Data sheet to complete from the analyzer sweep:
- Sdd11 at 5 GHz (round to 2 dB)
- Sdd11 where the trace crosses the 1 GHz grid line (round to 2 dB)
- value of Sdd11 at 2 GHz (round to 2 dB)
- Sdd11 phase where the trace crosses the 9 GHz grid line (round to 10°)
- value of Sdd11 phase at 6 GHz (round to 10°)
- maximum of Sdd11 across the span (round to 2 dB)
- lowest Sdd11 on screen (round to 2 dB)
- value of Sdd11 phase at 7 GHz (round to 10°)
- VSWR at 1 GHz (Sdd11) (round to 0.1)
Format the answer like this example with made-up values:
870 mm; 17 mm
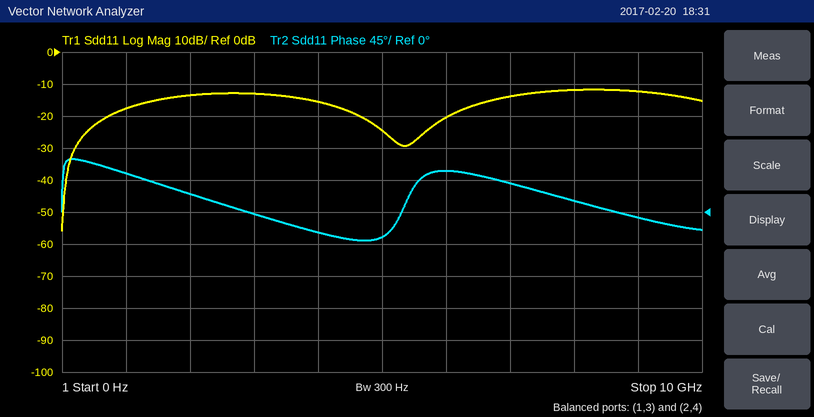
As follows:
-24 dB; -18 dB; -14 dB; -10°; 60°; -12 dB; -56 dB; 40°; 1.3
